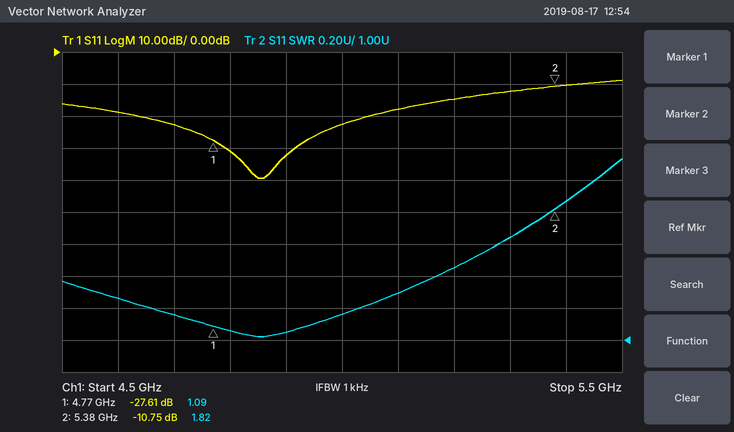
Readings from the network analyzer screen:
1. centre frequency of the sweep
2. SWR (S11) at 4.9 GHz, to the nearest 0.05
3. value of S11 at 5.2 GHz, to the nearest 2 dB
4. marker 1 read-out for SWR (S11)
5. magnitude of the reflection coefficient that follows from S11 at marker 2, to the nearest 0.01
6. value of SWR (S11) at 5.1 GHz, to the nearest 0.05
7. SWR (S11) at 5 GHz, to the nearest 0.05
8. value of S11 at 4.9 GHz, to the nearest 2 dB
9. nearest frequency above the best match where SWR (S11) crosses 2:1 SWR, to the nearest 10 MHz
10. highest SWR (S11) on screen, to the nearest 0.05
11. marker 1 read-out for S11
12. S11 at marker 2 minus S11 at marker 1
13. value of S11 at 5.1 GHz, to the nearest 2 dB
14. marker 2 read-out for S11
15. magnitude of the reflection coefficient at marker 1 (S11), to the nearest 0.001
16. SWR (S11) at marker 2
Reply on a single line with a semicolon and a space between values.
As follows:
5 GHz; 1.05; -14 dB; 1.09; 0.29; 1.30; 1.15; -32 dB; 5.45 GHz; 2.15; -27.61 dB; 16.86 dB; -18 dB; -10.75 dB; 0.042; 1.82
